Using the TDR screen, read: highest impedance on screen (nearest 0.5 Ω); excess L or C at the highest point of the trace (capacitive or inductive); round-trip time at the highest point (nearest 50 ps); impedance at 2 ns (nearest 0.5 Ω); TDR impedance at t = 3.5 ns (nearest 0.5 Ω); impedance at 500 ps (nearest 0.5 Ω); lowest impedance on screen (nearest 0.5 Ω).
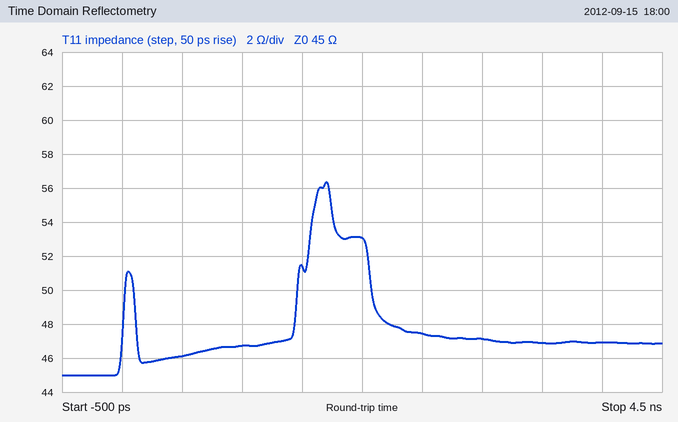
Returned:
56.5 Ω
inductive
1.70 ns
53.0 Ω
47.0 Ω
46.0 Ω
45.0 Ω
